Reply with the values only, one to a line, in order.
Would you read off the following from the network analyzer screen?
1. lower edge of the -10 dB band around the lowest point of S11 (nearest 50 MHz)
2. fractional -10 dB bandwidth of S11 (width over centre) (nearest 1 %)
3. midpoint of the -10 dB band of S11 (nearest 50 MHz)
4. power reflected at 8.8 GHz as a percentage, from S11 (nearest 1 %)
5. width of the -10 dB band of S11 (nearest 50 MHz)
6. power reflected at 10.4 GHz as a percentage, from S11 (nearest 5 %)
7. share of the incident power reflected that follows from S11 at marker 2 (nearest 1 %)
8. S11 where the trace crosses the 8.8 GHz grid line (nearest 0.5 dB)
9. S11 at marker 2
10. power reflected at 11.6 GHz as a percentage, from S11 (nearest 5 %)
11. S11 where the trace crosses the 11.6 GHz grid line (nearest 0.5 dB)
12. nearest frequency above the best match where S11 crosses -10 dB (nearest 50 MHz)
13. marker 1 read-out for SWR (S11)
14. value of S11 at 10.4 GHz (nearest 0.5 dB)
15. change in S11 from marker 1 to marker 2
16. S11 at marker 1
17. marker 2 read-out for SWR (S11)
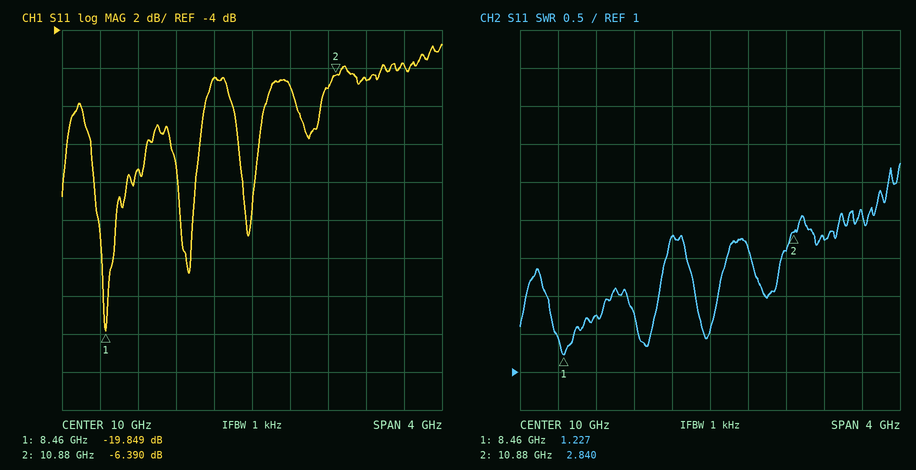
8.30 GHz
7 %
8.60 GHz
7 %
600 MHz
20 %
23 %
-11.5 dB
-6.390 dB
25 %
-6.0 dB
8.90 GHz
1.227
-7.0 dB
13.459 dB
-19.849 dB
2.840
